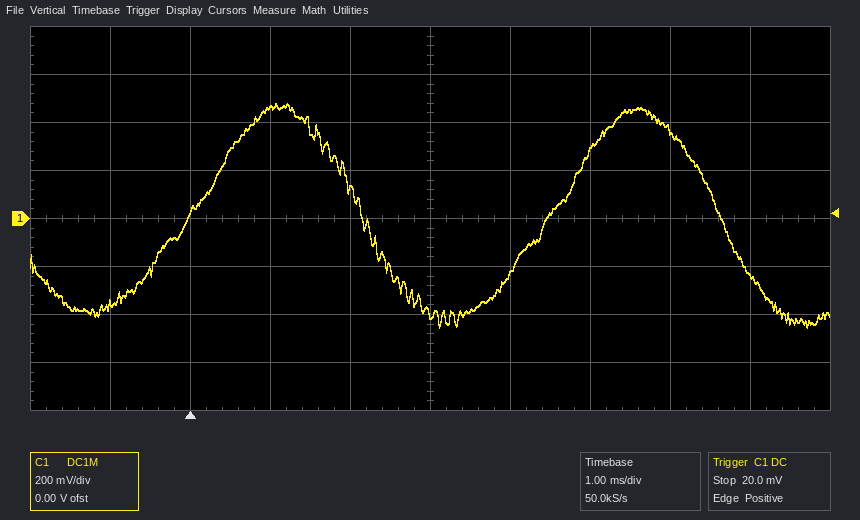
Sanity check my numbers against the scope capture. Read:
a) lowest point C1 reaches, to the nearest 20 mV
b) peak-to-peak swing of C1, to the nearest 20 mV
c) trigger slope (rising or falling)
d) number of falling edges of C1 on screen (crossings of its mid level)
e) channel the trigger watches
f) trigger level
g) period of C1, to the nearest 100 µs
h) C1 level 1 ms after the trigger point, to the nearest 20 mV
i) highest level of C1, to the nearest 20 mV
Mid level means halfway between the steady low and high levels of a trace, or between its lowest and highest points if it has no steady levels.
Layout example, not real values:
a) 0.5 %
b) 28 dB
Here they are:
a) -460 mV
b) 940 mV
c) rising
d) 2
e) C1
f) 20.0 mV
g) 4.5 ms
h) 460 mV
i) 480 mV
